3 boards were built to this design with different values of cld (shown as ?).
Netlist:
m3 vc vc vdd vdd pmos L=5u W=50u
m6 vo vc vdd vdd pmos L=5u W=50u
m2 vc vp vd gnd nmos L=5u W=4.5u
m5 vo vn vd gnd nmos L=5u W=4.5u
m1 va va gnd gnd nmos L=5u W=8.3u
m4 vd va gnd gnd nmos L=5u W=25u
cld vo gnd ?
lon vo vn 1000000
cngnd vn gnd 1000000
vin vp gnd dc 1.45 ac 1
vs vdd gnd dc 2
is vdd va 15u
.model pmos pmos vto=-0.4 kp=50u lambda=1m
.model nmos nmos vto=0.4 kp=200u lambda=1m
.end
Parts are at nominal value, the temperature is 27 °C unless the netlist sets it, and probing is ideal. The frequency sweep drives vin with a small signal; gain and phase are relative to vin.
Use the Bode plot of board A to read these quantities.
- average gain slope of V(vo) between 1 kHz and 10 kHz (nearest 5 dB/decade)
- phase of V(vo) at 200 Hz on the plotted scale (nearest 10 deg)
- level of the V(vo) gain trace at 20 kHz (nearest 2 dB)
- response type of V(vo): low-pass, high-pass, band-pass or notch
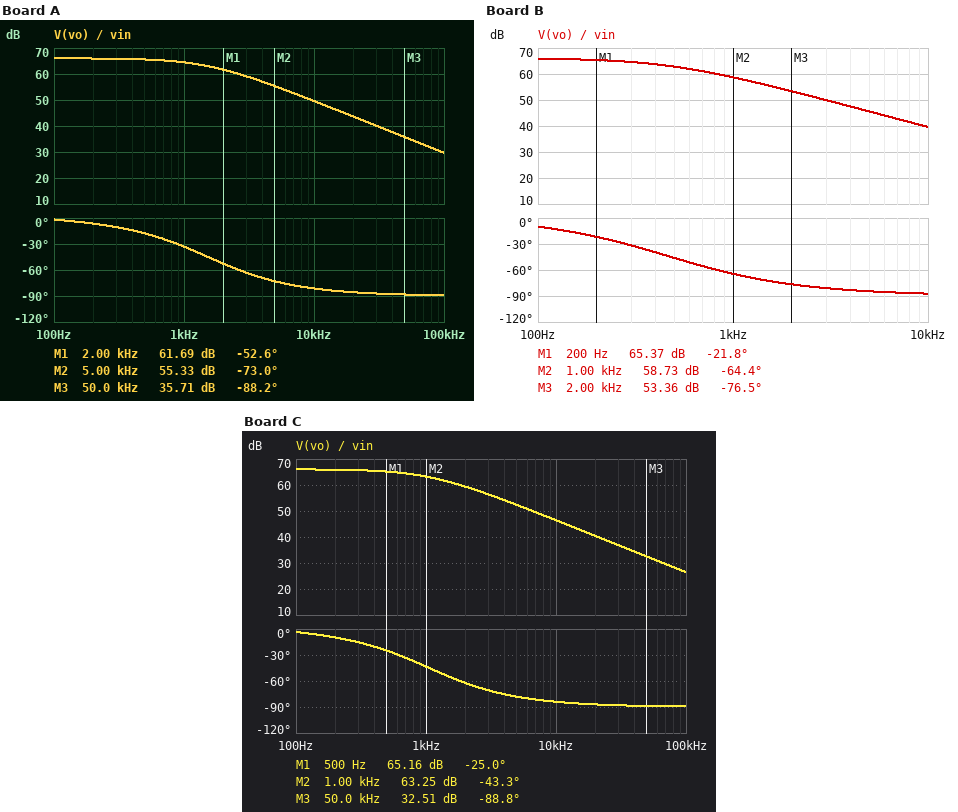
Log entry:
-15 dB/decade
-10 deg
44 dB
low-pass
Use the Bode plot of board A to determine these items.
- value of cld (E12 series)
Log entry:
4.7 pF
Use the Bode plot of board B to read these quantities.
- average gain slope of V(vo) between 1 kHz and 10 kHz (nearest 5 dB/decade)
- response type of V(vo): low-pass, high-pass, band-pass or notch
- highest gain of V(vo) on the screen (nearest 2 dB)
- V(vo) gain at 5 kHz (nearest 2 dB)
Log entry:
-20 dB/decade
low-pass
66 dB
46 dB
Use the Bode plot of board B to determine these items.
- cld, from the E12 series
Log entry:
15 pF
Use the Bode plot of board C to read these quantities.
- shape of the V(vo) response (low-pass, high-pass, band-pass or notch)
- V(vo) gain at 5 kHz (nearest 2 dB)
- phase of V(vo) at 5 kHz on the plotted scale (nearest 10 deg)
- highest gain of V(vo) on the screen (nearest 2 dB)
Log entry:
low-pass
52 dB
-80 deg
66 dB
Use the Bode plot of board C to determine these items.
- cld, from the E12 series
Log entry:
6.8 pF
